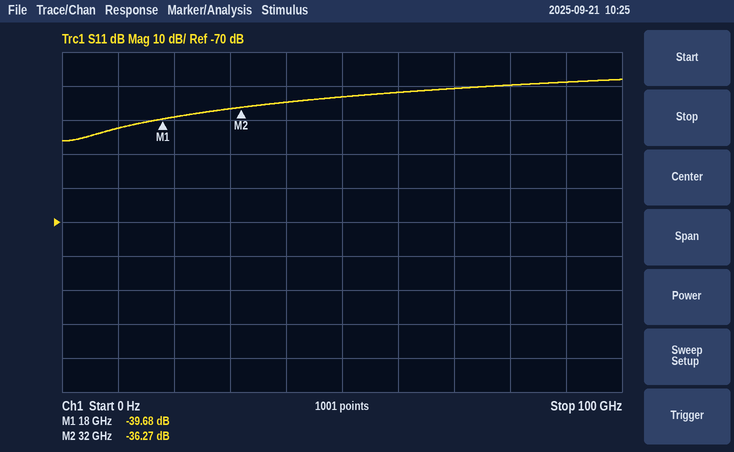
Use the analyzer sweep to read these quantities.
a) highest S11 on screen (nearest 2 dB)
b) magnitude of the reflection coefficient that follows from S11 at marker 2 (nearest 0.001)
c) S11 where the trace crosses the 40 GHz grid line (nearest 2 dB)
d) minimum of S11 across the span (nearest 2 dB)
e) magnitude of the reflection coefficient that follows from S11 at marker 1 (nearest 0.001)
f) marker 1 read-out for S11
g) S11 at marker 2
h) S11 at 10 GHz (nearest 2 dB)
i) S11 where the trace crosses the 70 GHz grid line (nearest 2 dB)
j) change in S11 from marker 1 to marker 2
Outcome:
-28 dB
0.015
-34 dB
-46 dB
0.010
-39.68 dB
-36.27 dB
-42 dB
-30 dB
3.41 dB
